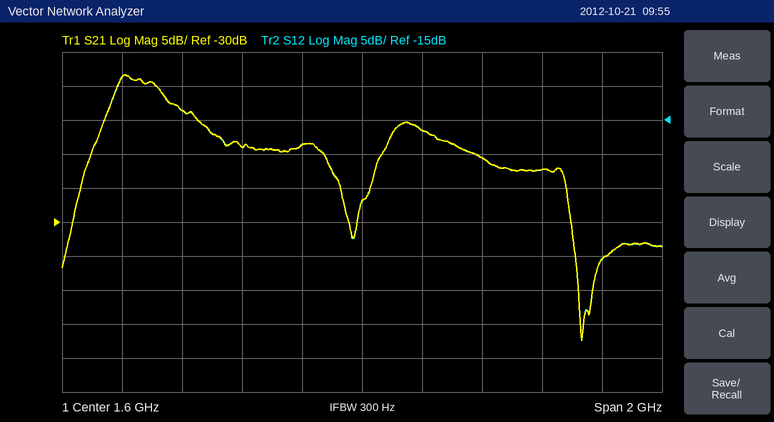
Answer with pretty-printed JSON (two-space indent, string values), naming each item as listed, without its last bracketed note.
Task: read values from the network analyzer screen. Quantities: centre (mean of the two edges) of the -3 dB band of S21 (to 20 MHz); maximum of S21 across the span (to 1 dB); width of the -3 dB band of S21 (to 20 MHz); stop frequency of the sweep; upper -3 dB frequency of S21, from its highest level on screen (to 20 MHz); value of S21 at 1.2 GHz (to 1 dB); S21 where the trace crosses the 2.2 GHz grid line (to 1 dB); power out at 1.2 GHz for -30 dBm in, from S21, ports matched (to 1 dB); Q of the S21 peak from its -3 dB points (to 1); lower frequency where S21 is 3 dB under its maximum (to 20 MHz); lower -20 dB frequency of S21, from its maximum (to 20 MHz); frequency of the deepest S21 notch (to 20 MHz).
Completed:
{
  "centre (mean of the two edges) of the -3 dB band of S21": "860 MHz",
  "maximum of S21 across the span": "-8 dB",
  "width of the -3 dB band of S21": "160 MHz",
  "stop frequency of the sweep": "2.6 GHz",
  "upper -3 dB frequency of S21, from its highest level on screen": "940 MHz",
  "value of S21 at 1.2 GHz": "-19 dB",
  "S21 where the trace crosses the 2.2 GHz grid line": "-22 dB",
  "power out at 1.2 GHz for -30 dBm in, from S21, ports matched": "-49 dBm",
  "Q of the S21 peak from its -3 dB points": "5",
  "lower frequency where S21 is 3 dB under its maximum": "780 MHz",
  "lower -20 dB frequency of S21, from its maximum": "640 MHz",
  "frequency of the deepest S21 notch": "2.34 GHz"
}
